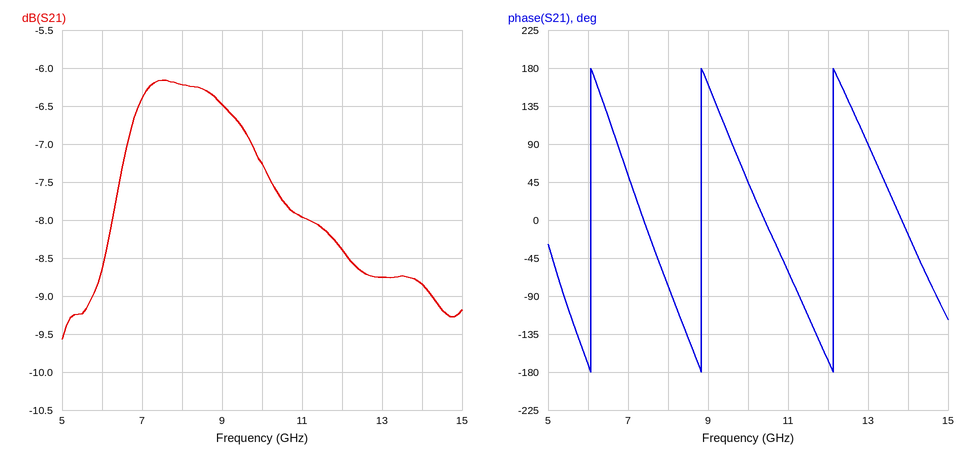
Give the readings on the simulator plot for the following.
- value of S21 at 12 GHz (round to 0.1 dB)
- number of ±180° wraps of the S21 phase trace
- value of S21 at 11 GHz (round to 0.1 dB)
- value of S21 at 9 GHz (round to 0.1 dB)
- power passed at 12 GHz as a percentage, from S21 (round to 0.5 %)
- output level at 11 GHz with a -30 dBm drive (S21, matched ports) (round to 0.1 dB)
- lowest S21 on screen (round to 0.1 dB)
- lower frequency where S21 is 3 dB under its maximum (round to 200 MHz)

-8.4 dB
3
-8.0 dB
-6.5 dB
14.5 %
-38.0 dBm
-9.6 dB
5.6 GHz
